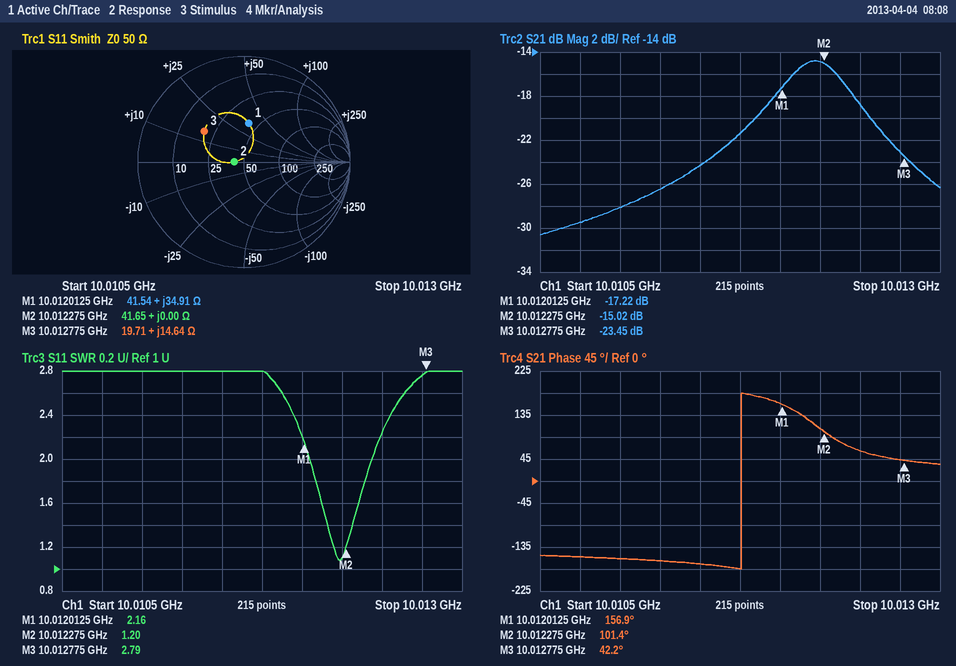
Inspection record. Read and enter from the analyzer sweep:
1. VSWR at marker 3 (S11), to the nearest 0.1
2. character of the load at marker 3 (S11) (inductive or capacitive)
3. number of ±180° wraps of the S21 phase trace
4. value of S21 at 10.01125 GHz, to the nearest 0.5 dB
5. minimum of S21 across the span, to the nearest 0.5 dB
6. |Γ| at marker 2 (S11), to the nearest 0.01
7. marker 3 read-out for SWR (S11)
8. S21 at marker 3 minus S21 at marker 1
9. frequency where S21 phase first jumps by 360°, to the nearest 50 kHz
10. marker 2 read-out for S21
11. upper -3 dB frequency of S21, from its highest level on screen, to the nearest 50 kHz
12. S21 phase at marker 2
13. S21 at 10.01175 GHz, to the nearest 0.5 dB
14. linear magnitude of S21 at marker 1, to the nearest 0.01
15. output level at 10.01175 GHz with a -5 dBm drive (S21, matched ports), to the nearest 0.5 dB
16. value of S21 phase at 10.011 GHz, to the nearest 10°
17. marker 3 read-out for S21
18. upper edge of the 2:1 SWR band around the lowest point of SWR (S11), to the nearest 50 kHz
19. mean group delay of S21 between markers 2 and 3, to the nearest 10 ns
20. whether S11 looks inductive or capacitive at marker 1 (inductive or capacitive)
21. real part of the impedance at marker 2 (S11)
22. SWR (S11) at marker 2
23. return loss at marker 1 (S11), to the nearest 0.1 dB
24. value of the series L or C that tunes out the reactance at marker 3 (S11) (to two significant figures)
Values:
2.8
inductive
1
-26.5 dB
-30.5 dB
0.09
2.79
-6.23 dB
10.01175 GHz
-15.02 dB
10.01245 GHz
101.4°
-21.5 dB
0.14
-26.5 dBm
-160°
-23.45 dB
10.01245 GHz
330 ns
inductive
41.65 Ω
1.20
8.7 dB
1.1 pF
